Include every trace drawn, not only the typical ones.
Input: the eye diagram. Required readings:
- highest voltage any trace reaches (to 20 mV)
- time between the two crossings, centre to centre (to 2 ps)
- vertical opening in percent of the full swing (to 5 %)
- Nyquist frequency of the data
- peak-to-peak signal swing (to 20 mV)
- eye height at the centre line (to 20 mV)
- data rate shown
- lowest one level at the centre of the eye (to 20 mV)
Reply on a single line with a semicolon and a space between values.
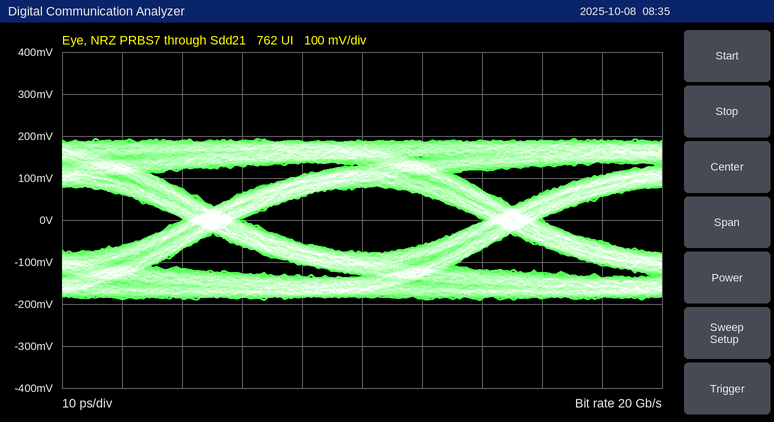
200 mV; 50 ps; 40 %; 10 GHz; 380 mV; 160 mV; 20 Gb/s; 80 mV
